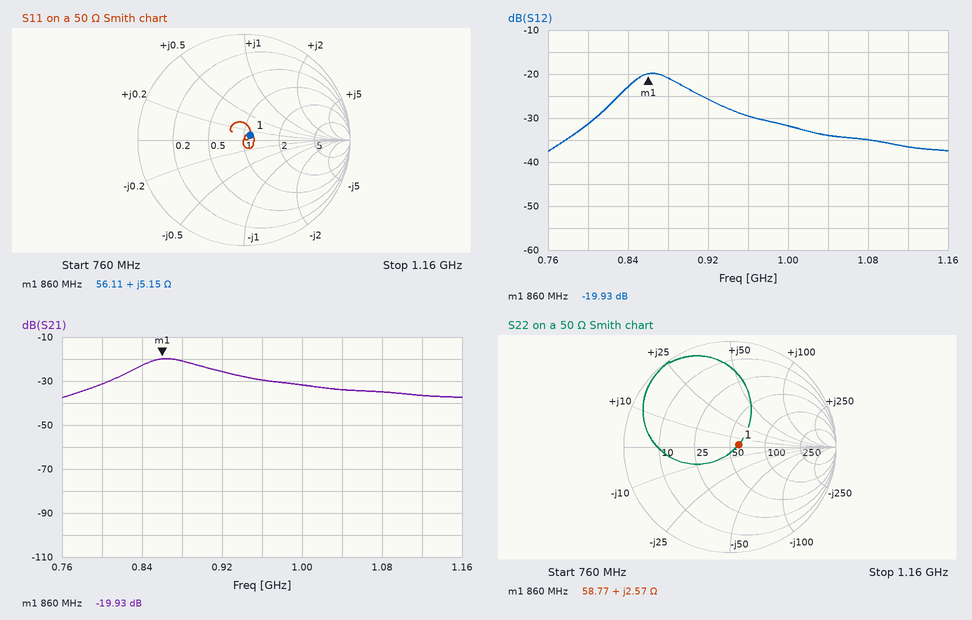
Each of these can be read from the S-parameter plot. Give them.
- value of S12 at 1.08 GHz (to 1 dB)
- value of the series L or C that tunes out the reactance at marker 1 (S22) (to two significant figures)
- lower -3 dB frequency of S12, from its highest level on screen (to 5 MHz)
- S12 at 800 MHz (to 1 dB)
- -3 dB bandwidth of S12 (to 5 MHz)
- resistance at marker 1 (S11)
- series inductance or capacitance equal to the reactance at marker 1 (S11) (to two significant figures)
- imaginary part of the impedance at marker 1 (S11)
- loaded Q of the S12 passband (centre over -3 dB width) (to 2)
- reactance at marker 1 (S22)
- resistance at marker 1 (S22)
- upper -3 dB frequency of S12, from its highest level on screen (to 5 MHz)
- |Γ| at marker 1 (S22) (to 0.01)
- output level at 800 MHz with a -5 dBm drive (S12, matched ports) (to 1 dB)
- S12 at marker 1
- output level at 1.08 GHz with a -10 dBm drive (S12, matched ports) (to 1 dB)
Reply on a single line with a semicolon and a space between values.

-35 dB; 72 pF; 840 MHz; -31 dB; 55 MHz; 56.11 Ω; 950 pH; +5.15 Ω; 16; +2.57 Ω; 58.77 Ω; 895 MHz; 0.08; -36 dBm; -19.93 dB; -45 dBm
